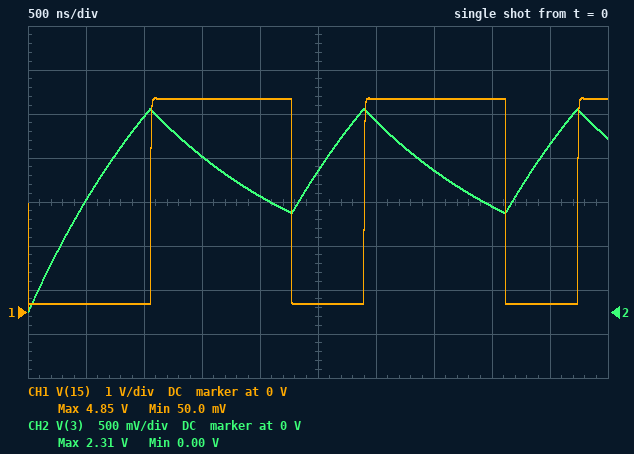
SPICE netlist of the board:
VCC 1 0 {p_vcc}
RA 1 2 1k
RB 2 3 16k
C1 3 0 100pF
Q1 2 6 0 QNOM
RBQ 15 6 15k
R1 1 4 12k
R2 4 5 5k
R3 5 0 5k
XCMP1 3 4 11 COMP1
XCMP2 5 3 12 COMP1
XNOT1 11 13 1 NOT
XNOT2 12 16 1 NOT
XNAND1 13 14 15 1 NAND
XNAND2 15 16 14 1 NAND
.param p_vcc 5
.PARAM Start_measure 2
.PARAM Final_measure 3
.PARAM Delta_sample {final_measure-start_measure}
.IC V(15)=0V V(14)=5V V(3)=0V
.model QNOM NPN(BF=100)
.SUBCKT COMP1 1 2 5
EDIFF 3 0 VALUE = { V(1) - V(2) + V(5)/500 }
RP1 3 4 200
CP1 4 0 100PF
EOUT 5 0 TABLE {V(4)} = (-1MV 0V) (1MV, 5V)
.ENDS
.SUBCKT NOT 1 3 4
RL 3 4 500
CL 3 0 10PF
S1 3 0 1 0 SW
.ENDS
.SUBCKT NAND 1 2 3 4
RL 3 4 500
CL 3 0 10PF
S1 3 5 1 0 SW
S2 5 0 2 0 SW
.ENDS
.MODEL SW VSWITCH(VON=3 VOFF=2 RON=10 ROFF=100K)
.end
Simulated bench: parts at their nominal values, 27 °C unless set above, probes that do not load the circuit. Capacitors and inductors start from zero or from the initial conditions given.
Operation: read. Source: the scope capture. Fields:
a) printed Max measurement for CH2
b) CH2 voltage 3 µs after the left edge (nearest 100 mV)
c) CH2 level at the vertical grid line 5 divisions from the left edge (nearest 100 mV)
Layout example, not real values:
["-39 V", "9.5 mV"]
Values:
["2.31 V", "2.2 V", "1.6 V"]
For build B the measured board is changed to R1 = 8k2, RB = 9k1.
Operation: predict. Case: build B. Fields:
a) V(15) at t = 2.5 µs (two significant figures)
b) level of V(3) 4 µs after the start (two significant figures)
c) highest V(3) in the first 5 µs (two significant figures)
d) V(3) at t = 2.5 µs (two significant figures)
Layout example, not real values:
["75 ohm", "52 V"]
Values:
["4.8 V", "1.5 V", "2.8 V", "1.7 V"]
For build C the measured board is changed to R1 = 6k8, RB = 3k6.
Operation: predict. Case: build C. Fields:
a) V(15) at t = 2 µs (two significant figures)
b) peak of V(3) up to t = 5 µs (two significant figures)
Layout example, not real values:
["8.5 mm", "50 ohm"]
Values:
["190 mV", "3.1 V"]
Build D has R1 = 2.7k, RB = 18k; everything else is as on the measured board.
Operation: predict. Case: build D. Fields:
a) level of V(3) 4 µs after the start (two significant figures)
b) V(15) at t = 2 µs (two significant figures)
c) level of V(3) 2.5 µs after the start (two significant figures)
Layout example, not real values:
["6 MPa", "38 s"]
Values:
["2.3 V", "190 mV", "3.7 V"]
